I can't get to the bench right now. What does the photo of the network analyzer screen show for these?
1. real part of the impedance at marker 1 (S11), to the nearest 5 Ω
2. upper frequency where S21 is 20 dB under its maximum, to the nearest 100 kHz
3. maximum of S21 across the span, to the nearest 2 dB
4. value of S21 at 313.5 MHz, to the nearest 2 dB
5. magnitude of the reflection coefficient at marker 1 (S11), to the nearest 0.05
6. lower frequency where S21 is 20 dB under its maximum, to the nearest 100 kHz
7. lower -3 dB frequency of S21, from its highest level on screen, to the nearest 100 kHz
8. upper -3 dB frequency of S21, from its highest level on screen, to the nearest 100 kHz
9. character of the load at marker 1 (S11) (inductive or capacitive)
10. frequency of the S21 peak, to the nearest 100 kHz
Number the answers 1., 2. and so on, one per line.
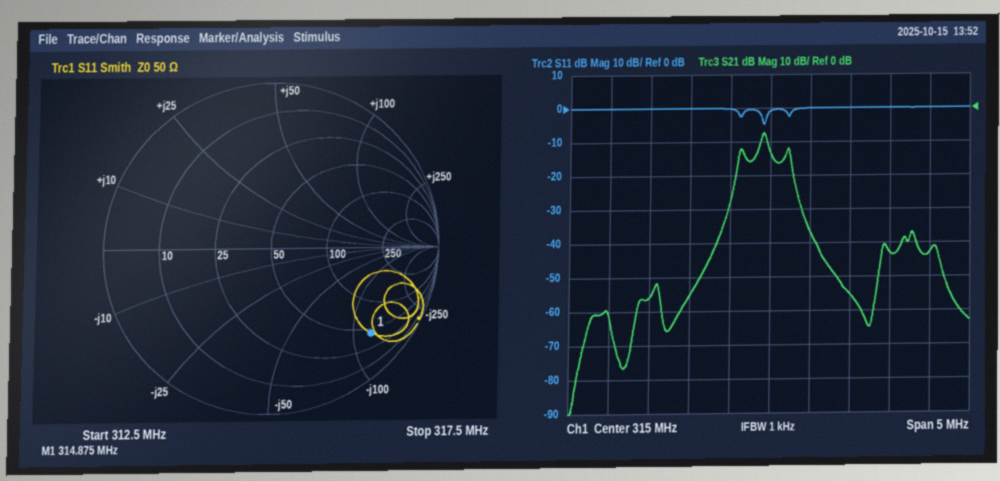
1. 45 Ω
2. 315.4 MHz
3. -8 dB
4. -56 dB
5. 0.80
6. 314.5 MHz
7. 314.9 MHz
8. 315.0 MHz
9. capacitive
10. 314.9 MHz
